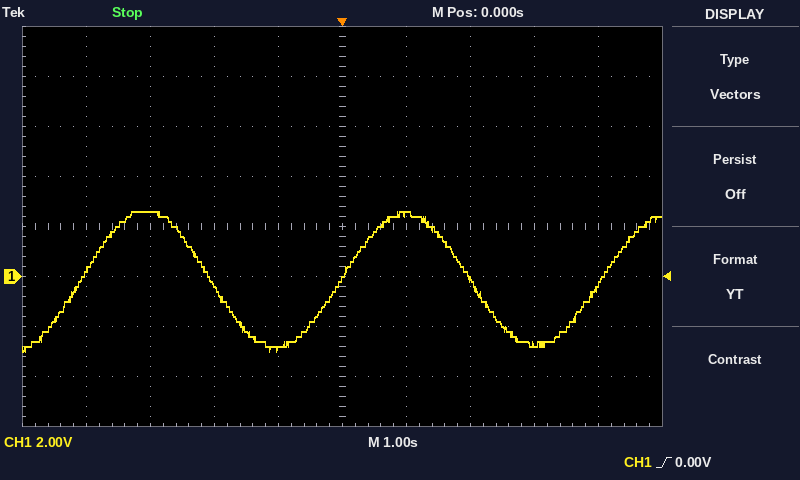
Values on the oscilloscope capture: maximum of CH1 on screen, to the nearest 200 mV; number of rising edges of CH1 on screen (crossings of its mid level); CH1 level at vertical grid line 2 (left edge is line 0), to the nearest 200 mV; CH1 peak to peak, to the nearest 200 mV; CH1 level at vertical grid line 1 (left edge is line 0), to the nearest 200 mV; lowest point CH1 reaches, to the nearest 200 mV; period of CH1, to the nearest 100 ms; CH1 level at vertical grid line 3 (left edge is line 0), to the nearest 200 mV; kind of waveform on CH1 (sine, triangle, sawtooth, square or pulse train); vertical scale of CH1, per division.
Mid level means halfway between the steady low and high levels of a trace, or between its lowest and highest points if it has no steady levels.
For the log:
2.6 V
3
2.6 V
5.6 V
200 mV
-3.0 V
4.1 s
-400 mV
sine
2 V
